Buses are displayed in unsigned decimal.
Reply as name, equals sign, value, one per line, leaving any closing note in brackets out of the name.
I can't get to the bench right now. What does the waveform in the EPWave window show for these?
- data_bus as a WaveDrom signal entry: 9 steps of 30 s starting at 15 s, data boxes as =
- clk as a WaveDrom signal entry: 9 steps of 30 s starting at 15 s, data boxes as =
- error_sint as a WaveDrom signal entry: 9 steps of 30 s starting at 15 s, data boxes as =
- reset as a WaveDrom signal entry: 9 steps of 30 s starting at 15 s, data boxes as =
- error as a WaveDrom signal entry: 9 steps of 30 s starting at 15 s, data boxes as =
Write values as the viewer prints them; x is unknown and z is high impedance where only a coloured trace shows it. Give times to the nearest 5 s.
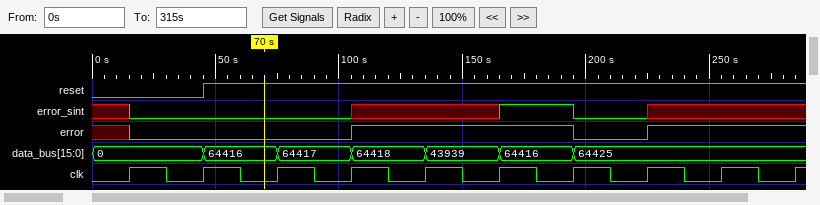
data_bus as a WaveDrom signal entry: 9 steps of 30 s starting at 15 s, data boxes as = = {name: 'data_bus', wave: '=======..', data: '0 64416 64417 64418 43939 64416 64425'}
clk as a WaveDrom signal entry: 9 steps of 30 s starting at 15 s, data boxes as = = {name: 'clk', wave: 'p........'}
error_sint as a WaveDrom signal entry: 9 steps of 30 s starting at 15 s, data boxes as = = {name: 'error_sint', wave: '0..x.10x.'}
reset as a WaveDrom signal entry: 9 steps of 30 s starting at 15 s, data boxes as = = {name: 'reset', wave: '01.......'}
error as a WaveDrom signal entry: 9 steps of 30 s starting at 15 s, data boxes as = = {name: 'error', wave: '0..1..01.'}
